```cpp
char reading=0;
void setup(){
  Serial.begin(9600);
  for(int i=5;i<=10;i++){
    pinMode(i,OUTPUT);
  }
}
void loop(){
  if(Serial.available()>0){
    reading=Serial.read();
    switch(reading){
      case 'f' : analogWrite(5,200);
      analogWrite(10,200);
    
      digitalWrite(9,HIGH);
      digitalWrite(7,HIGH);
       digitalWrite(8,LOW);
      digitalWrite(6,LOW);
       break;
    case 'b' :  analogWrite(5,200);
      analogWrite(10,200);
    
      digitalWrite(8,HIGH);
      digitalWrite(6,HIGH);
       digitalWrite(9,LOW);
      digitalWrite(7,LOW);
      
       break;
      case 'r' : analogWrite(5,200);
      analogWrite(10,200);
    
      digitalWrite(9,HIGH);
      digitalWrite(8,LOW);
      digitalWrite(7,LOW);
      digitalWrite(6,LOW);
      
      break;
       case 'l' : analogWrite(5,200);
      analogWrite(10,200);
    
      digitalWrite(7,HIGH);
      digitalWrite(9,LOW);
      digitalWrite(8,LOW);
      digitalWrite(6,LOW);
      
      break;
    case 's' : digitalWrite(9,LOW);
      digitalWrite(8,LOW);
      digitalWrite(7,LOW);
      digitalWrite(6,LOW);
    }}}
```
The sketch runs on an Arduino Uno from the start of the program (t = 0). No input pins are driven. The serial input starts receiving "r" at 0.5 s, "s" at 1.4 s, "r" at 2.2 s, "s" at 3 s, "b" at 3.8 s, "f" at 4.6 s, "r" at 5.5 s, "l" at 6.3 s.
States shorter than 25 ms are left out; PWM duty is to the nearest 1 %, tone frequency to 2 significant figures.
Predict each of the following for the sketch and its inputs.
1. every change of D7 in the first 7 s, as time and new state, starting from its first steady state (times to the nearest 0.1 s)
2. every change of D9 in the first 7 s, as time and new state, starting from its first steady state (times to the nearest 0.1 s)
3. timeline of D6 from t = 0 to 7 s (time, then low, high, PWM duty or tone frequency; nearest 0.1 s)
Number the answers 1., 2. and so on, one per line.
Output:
1. 0 s low; 4.6 s high; 5.5 s low; 6.3 s high
2. 0 s low; 0.5 s high; 1.4 s low; 2.2 s high; 3 s low; 4.6 s high; 6.3 s low
3. 0 s low; 3.8 s high; 4.6 s low
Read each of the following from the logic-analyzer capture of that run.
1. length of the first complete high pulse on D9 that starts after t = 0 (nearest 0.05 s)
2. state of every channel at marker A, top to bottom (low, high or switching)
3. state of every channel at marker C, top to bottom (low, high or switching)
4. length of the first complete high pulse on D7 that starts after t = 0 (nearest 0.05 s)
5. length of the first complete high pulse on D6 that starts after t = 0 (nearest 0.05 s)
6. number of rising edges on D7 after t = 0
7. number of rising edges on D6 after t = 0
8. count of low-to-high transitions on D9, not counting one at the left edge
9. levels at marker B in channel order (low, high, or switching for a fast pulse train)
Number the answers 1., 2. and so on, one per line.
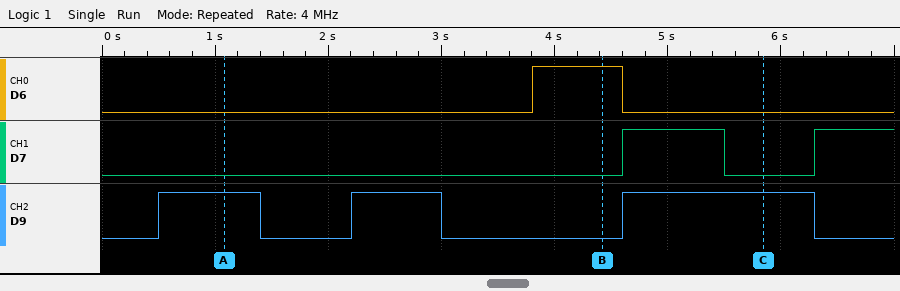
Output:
1. 0.90 s
2. D6 low, D7 low, D9 high
3. D6 low, D7 low, D9 high
4. 0.90 s
5. 0.80 s
6. 2
7. 1
8. 3
9. D6 high, D7 low, D9 low
